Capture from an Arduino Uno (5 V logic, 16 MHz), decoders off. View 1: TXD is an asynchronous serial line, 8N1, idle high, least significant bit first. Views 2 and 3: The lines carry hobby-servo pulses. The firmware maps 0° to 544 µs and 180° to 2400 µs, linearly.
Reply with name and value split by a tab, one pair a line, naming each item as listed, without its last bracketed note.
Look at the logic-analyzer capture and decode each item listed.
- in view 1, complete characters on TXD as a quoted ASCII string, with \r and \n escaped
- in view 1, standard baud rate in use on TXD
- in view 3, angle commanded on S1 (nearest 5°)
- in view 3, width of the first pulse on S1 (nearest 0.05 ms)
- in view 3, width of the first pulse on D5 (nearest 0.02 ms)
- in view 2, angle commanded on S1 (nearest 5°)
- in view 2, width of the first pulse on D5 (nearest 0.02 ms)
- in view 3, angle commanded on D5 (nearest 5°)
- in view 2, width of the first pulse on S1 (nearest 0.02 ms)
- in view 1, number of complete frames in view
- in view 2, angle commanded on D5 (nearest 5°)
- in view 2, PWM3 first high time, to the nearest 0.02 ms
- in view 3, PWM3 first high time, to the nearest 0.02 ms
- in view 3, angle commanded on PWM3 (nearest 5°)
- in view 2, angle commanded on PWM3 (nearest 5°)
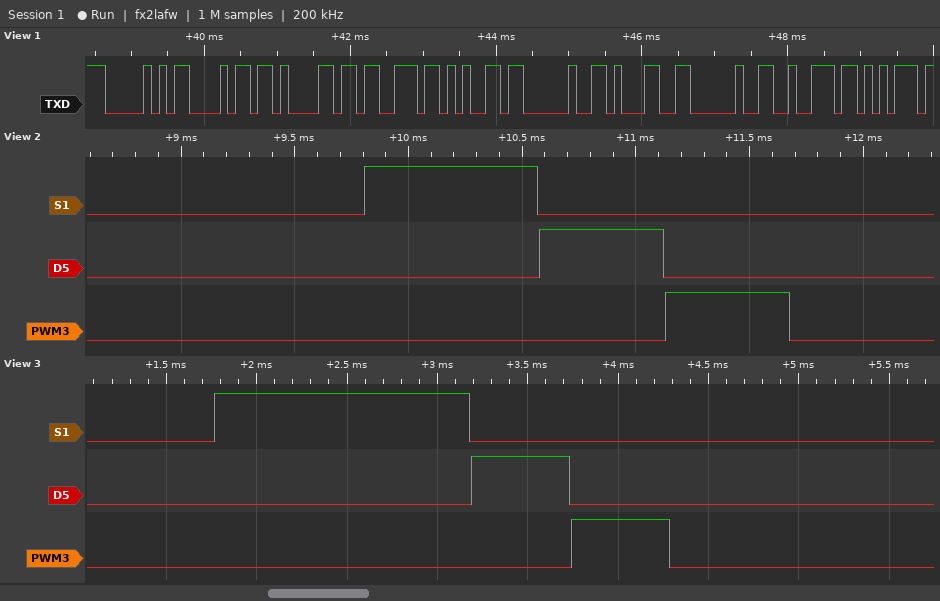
in view 1, complete characters on TXD as a quoted ASCII string, with \r and \n escaped	"Phase 1 ru"
in view 1, standard baud rate in use on TXD	9600 baud
in view 3, angle commanded on S1	85°
in view 3, width of the first pulse on S1	1.40 ms
in view 3, width of the first pulse on D5	0.54 ms
in view 2, angle commanded on S1	20°
in view 2, width of the first pulse on D5	0.54 ms
in view 3, angle commanded on D5	0°
in view 2, width of the first pulse on S1	0.76 ms
in view 1, number of complete frames in view	10
in view 2, angle commanded on D5	0°
in view 2, PWM3 first high time, to the nearest 0.02 ms	0.54 ms
in view 3, PWM3 first high time, to the nearest 0.02 ms	0.54 ms
in view 3, angle commanded on PWM3	0°
in view 2, angle commanded on PWM3	0°
